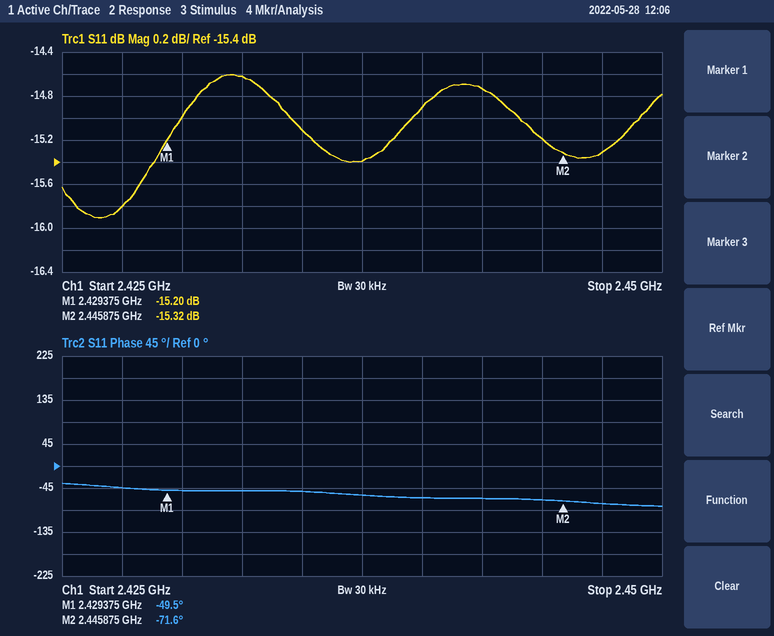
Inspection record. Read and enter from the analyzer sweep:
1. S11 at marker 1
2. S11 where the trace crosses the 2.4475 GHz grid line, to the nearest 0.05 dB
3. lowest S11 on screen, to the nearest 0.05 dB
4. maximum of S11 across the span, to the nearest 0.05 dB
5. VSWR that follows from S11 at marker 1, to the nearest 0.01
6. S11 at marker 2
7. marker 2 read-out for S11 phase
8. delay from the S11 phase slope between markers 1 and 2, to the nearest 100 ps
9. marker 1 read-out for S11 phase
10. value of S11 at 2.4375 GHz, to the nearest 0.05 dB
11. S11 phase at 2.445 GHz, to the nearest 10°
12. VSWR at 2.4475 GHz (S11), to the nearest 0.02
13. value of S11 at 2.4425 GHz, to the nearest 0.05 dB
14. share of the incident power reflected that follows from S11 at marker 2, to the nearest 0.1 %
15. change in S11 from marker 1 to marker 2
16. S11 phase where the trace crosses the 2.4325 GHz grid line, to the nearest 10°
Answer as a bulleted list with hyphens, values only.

- -15.20 dB
- -15.30 dB
- -15.90 dB
- -14.60 dB
- 1.42
- -15.32 dB
- -71.6°
- 3.7 ns
- -49.5°
- -15.40 dB
- -70°
- 1.42
- -14.75 dB
- 2.9 %
- -0.12 dB
- -50°
